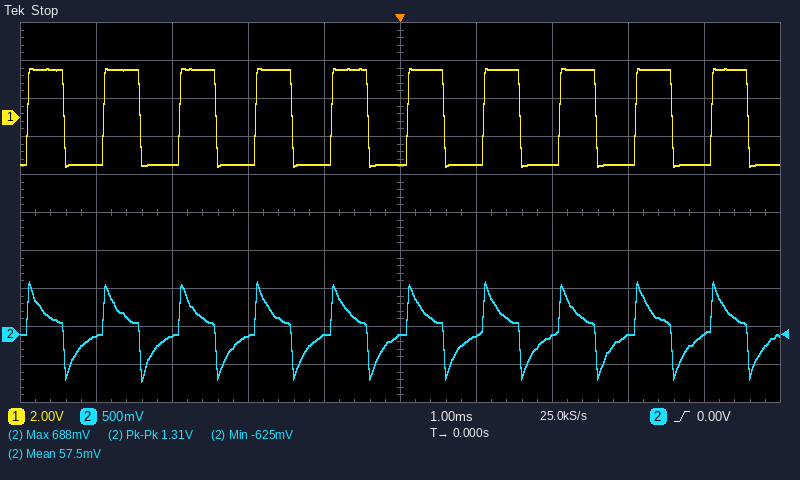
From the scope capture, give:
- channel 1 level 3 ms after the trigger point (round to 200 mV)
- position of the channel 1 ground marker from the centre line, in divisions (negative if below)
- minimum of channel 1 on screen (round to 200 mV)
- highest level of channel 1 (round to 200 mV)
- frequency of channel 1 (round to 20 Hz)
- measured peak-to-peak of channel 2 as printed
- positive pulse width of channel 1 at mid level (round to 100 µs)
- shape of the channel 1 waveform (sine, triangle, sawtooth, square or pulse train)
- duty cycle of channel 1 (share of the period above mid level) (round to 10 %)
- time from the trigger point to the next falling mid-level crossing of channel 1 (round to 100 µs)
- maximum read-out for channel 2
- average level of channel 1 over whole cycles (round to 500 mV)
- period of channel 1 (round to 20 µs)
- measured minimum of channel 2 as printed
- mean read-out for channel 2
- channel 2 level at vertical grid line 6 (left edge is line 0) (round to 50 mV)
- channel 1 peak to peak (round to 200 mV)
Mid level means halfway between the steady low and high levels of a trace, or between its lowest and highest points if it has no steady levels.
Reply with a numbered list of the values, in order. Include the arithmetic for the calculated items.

1. -2.4 V
2. +2.5 div
3. -2.6 V
4. 2.6 V
5. 1 / 1.00 ms ≈ 1.00 kHz
6. 1.31 V
7. 500 µs
8. square
9. 500 µs / 1.00 ms ≈ 50 %
10. 600 µs
11. 688 mV
12. -2.6 V + 0.5 × (2.6 V − (-2.6 V)) ≈ 0.0 V
13. 1.00 ms
14. -625 mV
15. 57.5 mV
16. 0 mV
17. 2.6 V − (-2.6 V) = 5.2 V
